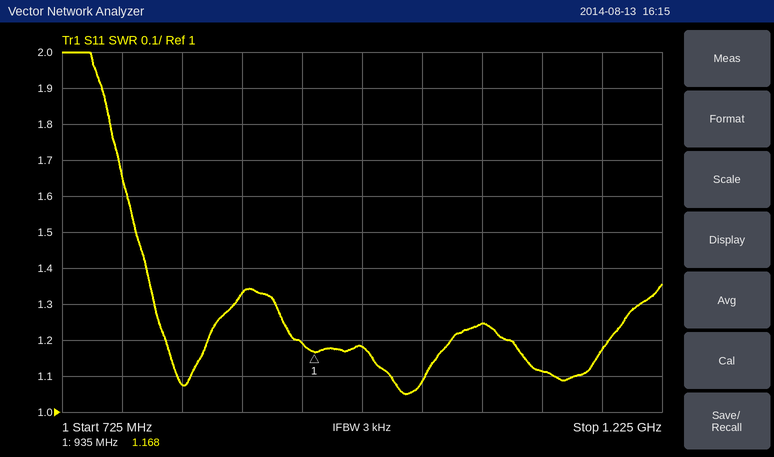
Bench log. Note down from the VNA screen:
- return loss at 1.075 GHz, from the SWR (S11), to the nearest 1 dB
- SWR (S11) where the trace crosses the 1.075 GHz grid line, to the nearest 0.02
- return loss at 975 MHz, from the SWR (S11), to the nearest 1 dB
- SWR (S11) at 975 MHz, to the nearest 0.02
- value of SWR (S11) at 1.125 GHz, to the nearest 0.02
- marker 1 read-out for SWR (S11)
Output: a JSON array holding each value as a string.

["19 dB", "1.24", "22 dB", "1.18", "1.12", "1.168"]
